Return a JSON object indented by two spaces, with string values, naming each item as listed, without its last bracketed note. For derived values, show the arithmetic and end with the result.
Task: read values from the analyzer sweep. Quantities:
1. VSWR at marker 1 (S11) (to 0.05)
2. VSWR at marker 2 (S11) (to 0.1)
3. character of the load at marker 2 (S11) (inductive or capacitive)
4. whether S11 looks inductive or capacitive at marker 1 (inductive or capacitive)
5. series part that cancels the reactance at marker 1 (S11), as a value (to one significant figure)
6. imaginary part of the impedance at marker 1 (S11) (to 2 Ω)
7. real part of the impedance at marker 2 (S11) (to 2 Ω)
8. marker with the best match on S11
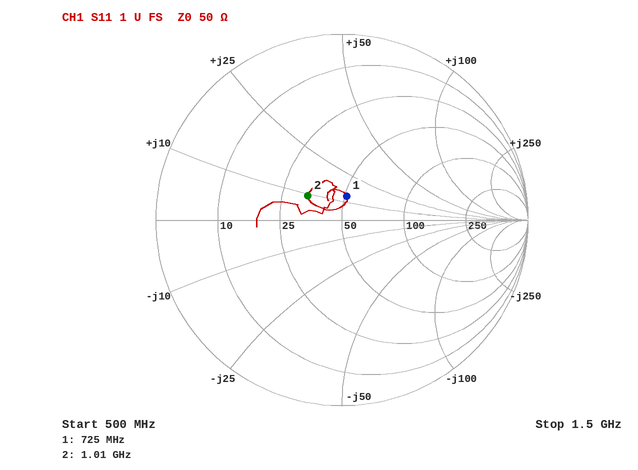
{
  "VSWR at marker 1 (S11)": "1.30",
  "VSWR at marker 2 (S11)": "1.6",
  "character of the load at marker 2 (S11)": "inductive",
  "whether S11 looks inductive or capacitive at marker 1": "inductive",
  "series part that cancels the reactance at marker 1 (S11), as a value": "C = 1/(2π × 725 MHz × 14 Ω) ≈ 15.7 pF, so 20 pF to one significant figure",
  "imaginary part of the impedance at marker 1 (S11)": "+14 Ω",
  "real part of the impedance at marker 2 (S11)": "34 Ω",
  "marker with the best match on S11": "marker 1"
}
